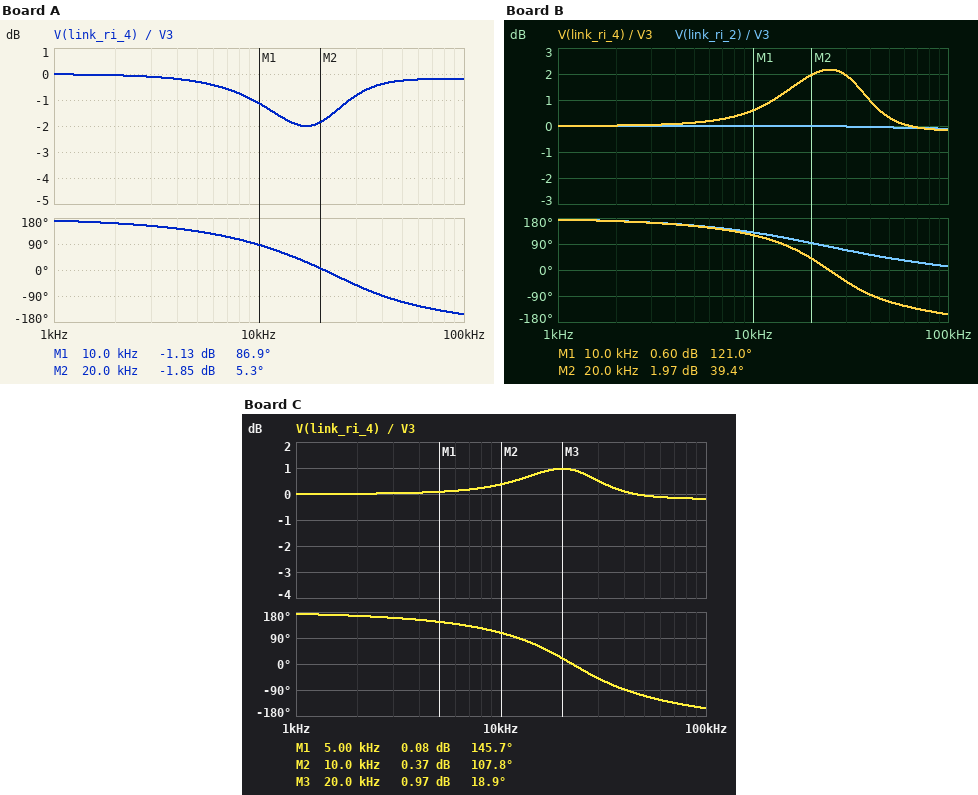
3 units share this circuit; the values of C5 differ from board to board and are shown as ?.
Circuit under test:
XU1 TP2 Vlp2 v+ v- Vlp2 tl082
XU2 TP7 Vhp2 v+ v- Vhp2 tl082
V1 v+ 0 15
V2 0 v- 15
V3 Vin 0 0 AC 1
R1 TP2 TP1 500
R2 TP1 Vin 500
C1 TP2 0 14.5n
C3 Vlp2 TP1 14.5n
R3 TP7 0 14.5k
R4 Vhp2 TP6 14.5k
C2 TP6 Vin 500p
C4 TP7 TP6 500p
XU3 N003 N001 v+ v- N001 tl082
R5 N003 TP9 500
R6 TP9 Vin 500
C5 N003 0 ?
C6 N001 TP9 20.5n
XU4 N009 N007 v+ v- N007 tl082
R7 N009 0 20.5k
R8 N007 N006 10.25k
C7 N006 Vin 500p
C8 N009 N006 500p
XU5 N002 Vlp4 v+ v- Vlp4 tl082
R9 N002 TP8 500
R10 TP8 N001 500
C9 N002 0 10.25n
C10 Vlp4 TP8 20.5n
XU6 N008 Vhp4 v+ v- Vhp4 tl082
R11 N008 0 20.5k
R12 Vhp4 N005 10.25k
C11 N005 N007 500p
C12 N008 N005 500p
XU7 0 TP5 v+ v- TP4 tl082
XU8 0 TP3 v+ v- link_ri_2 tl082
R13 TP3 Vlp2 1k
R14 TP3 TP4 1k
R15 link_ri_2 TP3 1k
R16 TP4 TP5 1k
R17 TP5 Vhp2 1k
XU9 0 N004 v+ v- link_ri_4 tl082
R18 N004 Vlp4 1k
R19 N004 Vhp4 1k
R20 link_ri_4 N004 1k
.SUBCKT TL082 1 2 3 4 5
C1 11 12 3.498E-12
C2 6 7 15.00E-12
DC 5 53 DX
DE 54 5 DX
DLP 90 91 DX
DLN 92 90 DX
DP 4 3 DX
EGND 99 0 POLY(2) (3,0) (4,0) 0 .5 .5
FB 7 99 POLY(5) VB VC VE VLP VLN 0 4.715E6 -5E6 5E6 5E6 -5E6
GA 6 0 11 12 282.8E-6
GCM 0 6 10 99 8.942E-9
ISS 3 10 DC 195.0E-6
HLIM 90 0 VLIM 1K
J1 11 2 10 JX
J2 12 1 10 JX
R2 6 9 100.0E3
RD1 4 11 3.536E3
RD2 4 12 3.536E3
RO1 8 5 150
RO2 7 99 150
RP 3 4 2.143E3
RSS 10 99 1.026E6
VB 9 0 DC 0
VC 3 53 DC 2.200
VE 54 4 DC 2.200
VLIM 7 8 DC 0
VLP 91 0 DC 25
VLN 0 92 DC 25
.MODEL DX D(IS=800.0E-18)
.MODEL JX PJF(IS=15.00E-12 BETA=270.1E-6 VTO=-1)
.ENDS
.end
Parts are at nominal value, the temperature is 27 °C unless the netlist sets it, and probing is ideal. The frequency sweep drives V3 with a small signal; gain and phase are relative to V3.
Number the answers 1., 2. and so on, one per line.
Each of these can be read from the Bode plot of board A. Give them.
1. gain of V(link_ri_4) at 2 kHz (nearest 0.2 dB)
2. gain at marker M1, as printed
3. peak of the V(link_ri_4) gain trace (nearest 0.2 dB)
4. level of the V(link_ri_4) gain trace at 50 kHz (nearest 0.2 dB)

1. 0 dB
2. -1.13 dB
3. 0 dB
4. -0.2 dB
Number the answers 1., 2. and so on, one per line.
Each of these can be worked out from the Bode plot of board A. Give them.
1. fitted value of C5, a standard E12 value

1. 15 nF
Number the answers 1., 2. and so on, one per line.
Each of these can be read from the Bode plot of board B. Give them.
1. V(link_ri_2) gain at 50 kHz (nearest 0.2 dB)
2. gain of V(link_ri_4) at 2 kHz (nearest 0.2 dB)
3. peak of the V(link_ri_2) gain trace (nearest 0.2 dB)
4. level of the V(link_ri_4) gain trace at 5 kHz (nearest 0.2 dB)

1. 0 dB
2. 0 dB
3. 0 dB
4. 0.2 dB
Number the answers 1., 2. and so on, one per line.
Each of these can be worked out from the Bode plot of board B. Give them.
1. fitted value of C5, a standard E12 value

1. 4.7 nF
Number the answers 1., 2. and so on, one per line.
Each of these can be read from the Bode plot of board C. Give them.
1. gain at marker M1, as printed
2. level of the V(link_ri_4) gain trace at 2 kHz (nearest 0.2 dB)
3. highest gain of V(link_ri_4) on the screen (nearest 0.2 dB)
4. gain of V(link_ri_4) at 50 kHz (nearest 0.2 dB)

1. 0.08 dB
2. 0 dB
3. 1.0 dB
4. 0 dB
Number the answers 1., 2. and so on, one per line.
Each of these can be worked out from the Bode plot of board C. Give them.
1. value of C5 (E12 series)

1. 8.2 nF
